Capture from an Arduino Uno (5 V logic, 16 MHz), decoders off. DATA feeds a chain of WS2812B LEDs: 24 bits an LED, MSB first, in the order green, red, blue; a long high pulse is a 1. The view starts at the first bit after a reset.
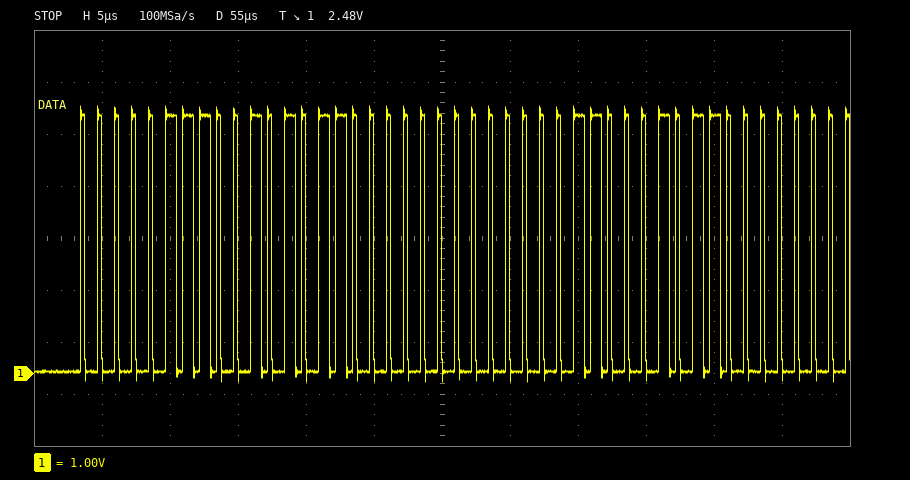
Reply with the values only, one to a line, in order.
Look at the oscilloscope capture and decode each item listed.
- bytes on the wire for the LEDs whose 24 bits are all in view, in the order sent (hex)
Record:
07 2B 00
